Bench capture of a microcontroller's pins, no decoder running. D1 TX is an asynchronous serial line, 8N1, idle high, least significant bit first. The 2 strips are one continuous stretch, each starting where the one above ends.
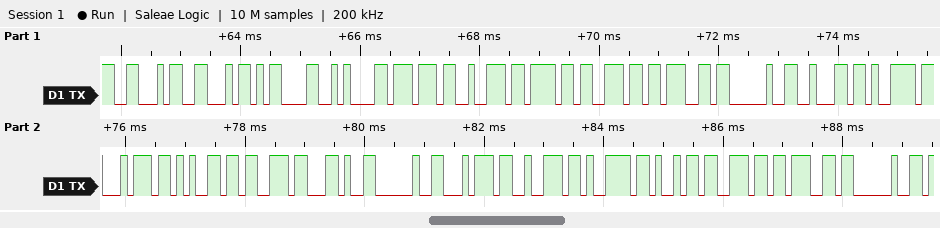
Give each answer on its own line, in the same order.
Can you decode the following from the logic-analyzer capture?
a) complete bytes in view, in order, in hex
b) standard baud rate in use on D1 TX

46 46 0D 0A 77 72 6F 6E 67 20 62 79 74 65 73 2C 20 74 72 79 69 6E 67 20
9600 baud
